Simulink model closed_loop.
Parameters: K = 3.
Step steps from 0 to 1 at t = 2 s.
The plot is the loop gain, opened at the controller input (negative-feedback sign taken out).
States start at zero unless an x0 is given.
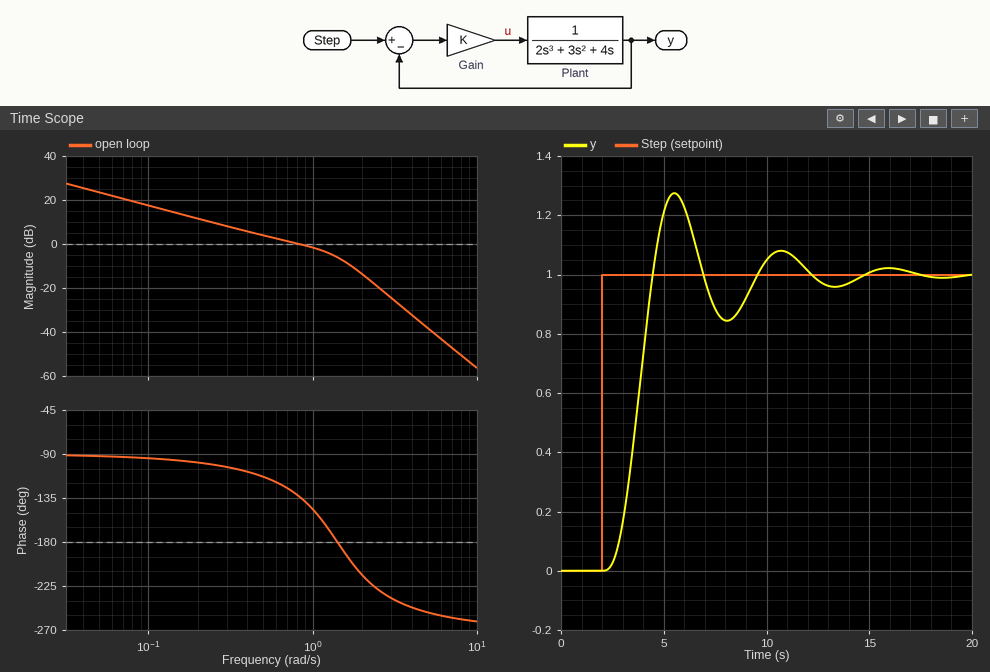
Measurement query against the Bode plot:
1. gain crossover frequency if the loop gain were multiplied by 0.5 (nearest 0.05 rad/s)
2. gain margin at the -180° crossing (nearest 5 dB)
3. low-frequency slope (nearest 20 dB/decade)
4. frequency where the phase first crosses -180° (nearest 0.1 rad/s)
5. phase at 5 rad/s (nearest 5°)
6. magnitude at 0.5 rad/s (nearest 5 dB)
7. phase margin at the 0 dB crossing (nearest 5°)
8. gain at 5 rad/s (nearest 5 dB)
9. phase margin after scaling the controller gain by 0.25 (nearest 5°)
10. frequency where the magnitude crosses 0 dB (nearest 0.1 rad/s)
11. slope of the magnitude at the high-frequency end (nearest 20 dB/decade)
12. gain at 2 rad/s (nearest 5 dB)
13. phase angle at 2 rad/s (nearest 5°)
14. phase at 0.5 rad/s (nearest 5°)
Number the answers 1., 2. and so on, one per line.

1. 0.40 rad/s
2. 5 dB
3. -20 dB/decade
4. 1.4 rad/s
5. -250°
6. 5 dB
7. 45°
8. -40 dB
9. 80°
10. 0.8 rad/s
11. -60 dB/decade
12. -15 dB
13. -215°
14. -115°
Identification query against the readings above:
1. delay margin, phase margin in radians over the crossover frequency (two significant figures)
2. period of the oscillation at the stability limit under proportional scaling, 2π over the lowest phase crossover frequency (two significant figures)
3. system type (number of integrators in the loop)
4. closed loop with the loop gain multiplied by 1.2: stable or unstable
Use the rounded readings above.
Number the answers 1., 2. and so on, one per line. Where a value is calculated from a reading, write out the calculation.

1. 45 × π / 180 / 0.8 = 0.98 s
2. 2π / 1.4 = 4.5 s
3. 1
4. stable
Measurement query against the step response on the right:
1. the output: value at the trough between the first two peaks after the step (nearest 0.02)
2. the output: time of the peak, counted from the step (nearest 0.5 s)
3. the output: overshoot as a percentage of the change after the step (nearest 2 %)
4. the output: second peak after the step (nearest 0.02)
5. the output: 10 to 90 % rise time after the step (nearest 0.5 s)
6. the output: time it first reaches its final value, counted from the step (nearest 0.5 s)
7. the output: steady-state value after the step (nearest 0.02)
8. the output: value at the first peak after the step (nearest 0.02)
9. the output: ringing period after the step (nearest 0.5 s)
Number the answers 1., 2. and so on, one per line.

1. 0.84
2. 3.5 s
3. 28 %
4. 1.08
5. 1.5 s
6. 2.5 s
7. 1.00
8. 1.28
9. 5.0 s
